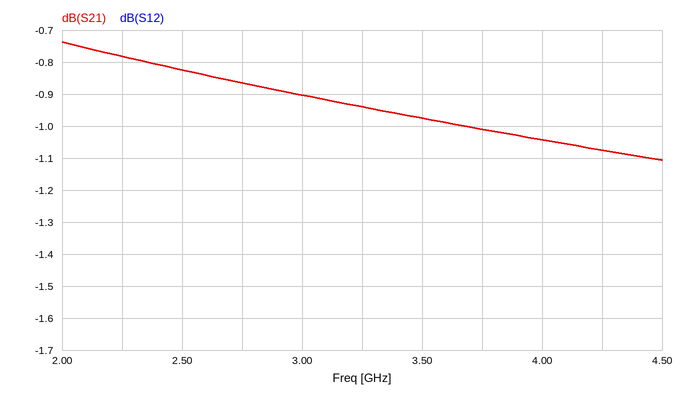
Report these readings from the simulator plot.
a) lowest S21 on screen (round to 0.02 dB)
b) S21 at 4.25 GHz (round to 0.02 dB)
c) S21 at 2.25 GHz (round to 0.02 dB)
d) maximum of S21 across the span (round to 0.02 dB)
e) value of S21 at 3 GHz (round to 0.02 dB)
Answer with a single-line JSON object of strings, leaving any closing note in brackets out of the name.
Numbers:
{"lowest S21 on screen": "-1.10 dB", "S21 at 4.25 GHz": "-1.08 dB", "S21 at 2.25 GHz": "-0.78 dB", "maximum of S21 across the span": "-0.74 dB", "value of S21 at 3 GHz": "-0.90 dB"}
